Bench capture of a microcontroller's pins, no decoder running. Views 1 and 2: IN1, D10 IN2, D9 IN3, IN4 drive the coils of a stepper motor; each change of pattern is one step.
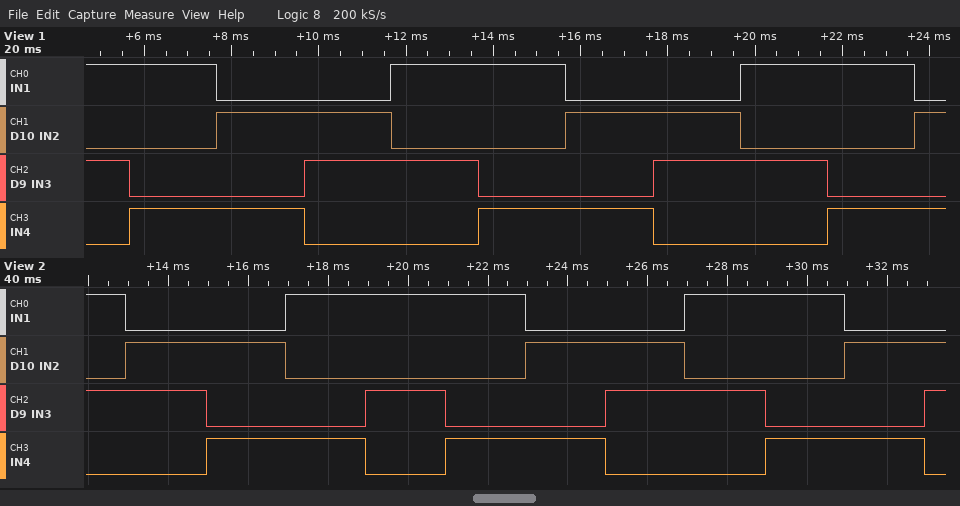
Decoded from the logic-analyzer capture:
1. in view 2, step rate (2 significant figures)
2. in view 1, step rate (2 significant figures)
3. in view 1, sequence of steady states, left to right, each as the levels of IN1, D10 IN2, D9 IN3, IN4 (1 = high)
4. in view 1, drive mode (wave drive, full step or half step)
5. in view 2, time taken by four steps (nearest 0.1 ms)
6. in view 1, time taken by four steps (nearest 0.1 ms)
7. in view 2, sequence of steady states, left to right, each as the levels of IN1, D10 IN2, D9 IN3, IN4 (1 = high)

500 steps/s
500 steps/s
1010 1001 0101 0110 1010 1001 0101 0110 1010 1001 0101
full step
8.0 ms
8.0 ms
1010 0110 0101 1001 1010 1001 0101 0110 1010 1001 0101 0110
